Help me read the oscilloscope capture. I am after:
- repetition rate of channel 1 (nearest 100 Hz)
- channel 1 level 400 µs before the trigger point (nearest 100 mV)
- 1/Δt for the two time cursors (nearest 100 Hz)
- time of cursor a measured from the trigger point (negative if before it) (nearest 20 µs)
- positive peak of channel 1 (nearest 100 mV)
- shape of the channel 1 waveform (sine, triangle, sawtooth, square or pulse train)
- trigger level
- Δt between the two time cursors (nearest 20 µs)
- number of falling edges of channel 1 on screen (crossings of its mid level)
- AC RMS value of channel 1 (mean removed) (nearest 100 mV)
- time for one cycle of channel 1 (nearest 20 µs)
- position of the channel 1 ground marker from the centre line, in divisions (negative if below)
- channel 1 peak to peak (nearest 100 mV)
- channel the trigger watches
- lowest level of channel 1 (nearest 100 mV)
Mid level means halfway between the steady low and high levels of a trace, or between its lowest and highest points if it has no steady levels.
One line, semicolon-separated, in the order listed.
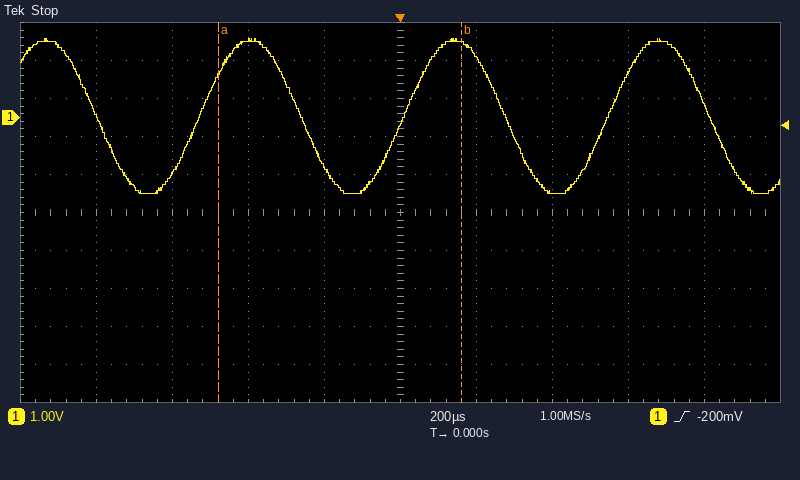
1.9 kHz; 2.0 V; 1.6 kHz; -480 µs; 2.1 V; sine; -200 mV; 640 µs; 4; 1.4 V; 540 µs; +2.5 div; 4.1 V; channel 1; -2.0 V
